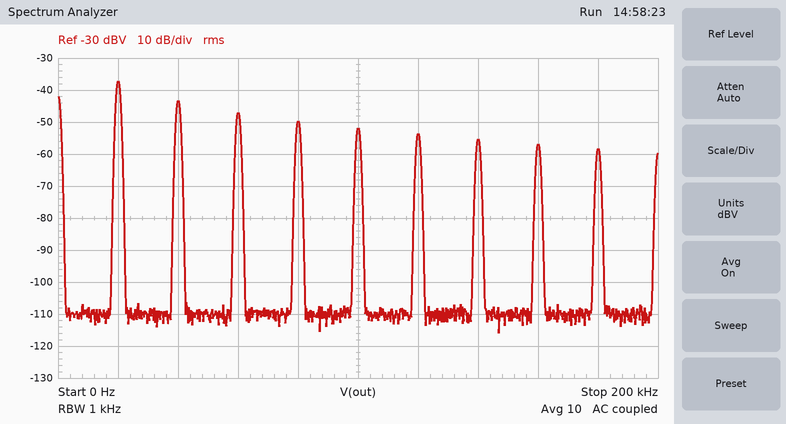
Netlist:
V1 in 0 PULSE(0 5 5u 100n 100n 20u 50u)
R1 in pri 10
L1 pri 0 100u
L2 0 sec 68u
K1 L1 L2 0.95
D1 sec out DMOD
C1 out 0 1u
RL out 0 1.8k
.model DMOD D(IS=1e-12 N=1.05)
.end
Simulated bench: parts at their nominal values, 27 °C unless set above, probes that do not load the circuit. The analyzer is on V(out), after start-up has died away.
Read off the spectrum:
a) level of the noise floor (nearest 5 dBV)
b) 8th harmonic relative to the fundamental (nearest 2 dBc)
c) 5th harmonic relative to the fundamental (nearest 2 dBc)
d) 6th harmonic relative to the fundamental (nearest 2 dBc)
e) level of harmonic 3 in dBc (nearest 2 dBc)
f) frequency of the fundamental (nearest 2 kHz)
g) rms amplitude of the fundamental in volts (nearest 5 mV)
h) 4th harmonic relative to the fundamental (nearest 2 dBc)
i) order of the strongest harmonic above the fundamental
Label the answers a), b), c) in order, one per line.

a) -110 dBV
b) -20 dBc
c) -14 dBc
d) -16 dBc
e) -10 dBc
f) 20 kHz
g) 15 mV
h) -12 dBc
i) 2
